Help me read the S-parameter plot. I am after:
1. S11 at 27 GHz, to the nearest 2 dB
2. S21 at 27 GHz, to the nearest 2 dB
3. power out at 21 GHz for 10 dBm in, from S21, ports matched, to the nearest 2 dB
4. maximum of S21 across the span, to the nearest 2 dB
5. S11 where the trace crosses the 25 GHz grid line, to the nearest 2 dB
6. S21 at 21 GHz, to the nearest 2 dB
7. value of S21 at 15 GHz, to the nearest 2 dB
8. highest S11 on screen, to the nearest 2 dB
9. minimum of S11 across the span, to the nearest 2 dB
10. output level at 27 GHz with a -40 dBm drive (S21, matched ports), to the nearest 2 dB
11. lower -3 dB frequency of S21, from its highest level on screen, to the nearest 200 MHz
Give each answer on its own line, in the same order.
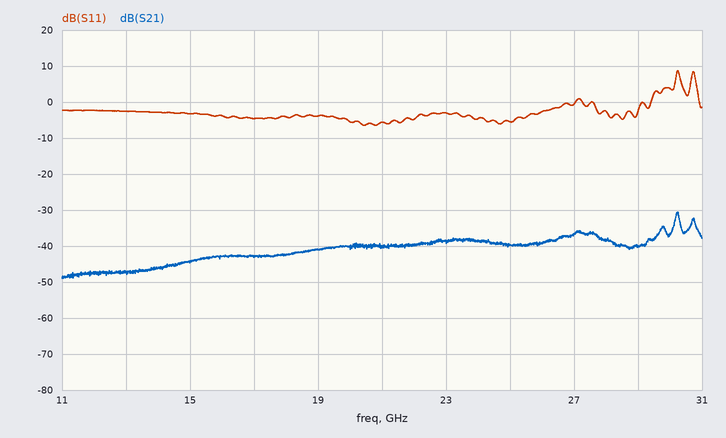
0 dB
-36 dB
-30 dBm
-30 dB
-6 dB
-40 dB
-44 dB
8 dB
-6 dB
-76 dBm
30.2 GHz
